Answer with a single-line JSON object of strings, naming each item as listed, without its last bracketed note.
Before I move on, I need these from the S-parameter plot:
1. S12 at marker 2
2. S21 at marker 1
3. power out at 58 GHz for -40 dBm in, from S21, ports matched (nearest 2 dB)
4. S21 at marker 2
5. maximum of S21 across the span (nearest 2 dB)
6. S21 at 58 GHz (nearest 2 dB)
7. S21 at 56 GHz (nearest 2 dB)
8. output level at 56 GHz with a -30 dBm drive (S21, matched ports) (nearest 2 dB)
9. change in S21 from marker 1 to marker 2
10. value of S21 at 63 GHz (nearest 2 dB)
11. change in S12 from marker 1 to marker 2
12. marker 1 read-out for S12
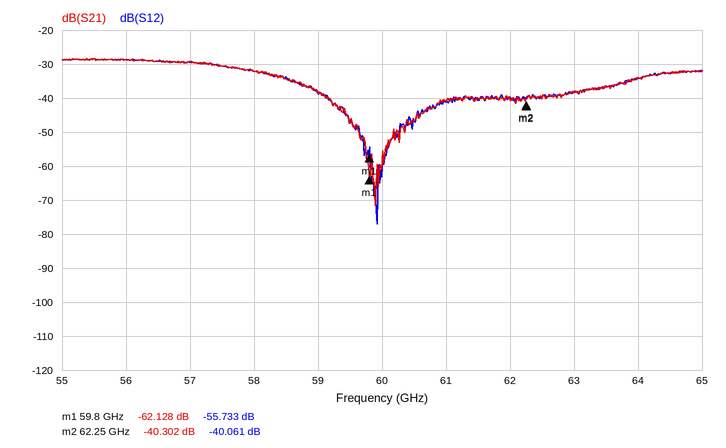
{"S12 at marker 2": "-40.061 dB", "S21 at marker 1": "-62.128 dB", "power out at 58 GHz for -40 dBm in, from S21, ports matched": "-72 dBm", "S21 at marker 2": "-40.302 dB", "maximum of S21 across the span": "-28 dB", "S21 at 58 GHz": "-32 dB", "S21 at 56 GHz": "-28 dB", "output level at 56 GHz with a -30 dBm drive (S21, matched ports)": "-58 dBm", "change in S21 from marker 1 to marker 2": "21.826 dB", "value of S21 at 63 GHz": "-38 dB", "change in S12 from marker 1 to marker 2": "15.672 dB", "marker 1 read-out for S12": "-55.733 dB"}
